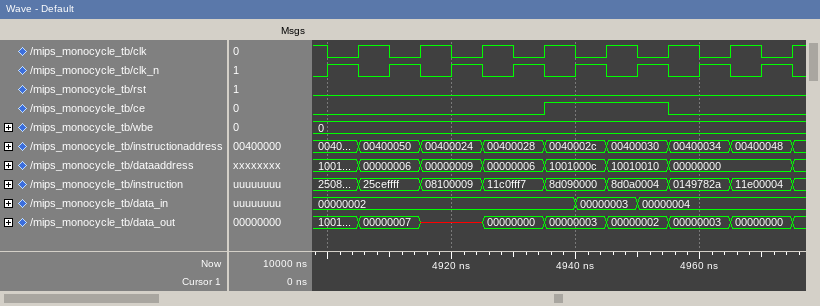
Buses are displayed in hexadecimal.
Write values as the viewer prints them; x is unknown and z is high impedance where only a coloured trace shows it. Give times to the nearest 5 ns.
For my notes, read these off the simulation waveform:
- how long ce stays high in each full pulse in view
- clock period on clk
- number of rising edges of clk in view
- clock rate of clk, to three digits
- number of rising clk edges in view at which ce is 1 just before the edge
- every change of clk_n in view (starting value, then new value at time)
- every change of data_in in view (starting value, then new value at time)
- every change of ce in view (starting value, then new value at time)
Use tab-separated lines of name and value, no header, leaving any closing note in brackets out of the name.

how long ce stays high in each full pulse in view	20 ns
clock period on clk	10 ns
number of rising edges of clk in view	8
clock rate of clk, to three digits	100 MHz
number of rising clk edges in view at which ce is 1 just before the edge	2
every change of clk_n in view	0, 1 at 4900 ns, 0 at 4905 ns, 1 at 4910 ns, 0 at 4915 ns, 1 at 4920 ns, 0 at 4925 ns, 1 at 4930 ns, 0 at 4935 ns, 1 at 4940 ns, 0 at 4945 ns, 1 at 4950 ns, 0 at 4955 ns, 1 at 4960 ns, 0 at 4965 ns, 1 at 4970 ns, 0 at 4975 ns
every change of data_in in view	00000002, 00000003 at 4940 ns, 00000004 at 4950 ns
every change of ce in view	0, 1 at 4935 ns, 0 at 4955 ns
